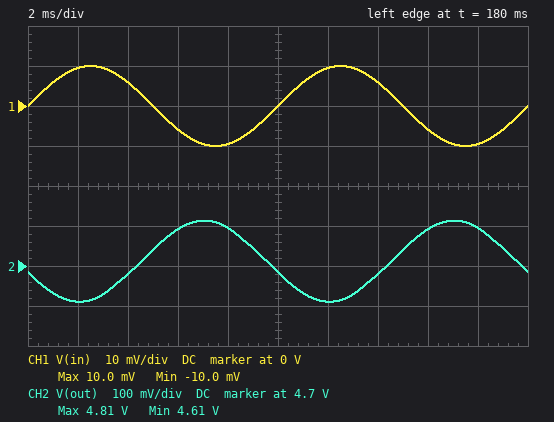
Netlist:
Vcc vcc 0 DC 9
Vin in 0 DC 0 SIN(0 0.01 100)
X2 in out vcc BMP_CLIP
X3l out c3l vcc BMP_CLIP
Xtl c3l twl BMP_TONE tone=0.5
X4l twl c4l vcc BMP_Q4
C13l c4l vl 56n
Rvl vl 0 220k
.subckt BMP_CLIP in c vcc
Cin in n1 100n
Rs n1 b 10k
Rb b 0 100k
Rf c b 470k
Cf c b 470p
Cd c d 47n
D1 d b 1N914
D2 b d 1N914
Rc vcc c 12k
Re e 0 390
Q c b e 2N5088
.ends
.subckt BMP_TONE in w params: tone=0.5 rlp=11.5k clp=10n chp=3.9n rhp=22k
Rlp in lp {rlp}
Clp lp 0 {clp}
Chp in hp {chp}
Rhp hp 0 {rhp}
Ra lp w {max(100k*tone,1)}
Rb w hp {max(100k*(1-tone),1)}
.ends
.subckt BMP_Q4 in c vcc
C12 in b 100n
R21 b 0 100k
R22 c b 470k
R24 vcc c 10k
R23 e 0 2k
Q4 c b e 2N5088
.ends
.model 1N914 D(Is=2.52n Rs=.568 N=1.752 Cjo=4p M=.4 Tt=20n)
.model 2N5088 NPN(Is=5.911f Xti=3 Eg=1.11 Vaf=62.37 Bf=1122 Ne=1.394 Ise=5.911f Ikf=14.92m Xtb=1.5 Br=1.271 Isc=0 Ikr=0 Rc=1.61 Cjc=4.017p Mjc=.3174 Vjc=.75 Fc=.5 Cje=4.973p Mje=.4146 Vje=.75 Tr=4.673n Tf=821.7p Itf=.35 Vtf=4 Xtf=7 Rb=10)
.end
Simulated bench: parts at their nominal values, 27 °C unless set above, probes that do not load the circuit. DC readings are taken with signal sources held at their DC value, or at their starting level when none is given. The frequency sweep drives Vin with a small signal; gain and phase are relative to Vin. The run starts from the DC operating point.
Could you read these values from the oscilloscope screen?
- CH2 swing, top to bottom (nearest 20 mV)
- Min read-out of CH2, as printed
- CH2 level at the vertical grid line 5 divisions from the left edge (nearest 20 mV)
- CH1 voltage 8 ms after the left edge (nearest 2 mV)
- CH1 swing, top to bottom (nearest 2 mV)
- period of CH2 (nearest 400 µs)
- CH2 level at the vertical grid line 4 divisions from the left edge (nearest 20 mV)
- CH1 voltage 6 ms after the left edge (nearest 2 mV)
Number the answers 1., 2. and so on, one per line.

1. 200 mV
2. 4.61 V
3. 4.68 V
4. -10 mV
5. 20 mV
6. 10.0 ms
7. 4.80 V
8. -6 mV
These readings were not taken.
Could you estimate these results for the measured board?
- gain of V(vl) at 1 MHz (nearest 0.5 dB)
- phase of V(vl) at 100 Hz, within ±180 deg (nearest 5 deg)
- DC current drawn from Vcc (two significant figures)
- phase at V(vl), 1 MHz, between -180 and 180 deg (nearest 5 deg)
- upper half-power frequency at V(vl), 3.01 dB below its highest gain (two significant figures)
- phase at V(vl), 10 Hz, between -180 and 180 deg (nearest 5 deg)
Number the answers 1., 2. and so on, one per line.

1. -53.5 dB
2. -115 deg
3. 970 µA
4. -165 deg
5. 790 Hz
6. 95 deg
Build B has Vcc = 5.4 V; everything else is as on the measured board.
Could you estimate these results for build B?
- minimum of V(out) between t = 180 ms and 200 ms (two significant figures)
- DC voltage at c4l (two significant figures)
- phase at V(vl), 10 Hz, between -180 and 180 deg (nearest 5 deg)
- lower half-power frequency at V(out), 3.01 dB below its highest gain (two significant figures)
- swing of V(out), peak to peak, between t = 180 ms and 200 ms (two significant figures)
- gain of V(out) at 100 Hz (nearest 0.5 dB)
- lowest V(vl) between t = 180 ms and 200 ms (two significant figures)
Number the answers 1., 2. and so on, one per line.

1. 3.8 V
2. 4.5 V
3. 90 deg
4. 38 Hz
5. 170 mV
6. 19.0 dB
7. -380 mV
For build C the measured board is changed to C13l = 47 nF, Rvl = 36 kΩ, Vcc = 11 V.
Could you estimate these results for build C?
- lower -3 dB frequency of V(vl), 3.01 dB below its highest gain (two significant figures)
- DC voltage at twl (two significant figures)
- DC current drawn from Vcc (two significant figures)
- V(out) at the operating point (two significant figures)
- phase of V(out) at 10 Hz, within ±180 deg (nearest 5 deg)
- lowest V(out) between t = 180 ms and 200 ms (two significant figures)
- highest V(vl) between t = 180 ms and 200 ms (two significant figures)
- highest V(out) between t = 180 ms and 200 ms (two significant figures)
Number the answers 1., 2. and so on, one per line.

1. 98 Hz
2. 2.7 V
3. 1.3 mA
4. 5.1 V
5. -100 deg
6. 5.0 V
7. 430 mV
8. 5.2 V
